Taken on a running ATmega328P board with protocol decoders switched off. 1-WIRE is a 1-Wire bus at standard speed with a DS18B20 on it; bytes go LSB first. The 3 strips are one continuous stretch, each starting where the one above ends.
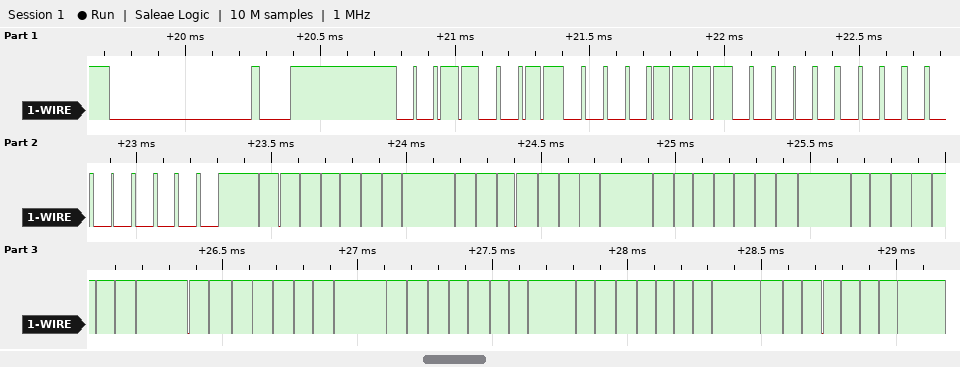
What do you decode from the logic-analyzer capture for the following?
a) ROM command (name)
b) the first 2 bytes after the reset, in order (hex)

Skip ROM
CC F0
